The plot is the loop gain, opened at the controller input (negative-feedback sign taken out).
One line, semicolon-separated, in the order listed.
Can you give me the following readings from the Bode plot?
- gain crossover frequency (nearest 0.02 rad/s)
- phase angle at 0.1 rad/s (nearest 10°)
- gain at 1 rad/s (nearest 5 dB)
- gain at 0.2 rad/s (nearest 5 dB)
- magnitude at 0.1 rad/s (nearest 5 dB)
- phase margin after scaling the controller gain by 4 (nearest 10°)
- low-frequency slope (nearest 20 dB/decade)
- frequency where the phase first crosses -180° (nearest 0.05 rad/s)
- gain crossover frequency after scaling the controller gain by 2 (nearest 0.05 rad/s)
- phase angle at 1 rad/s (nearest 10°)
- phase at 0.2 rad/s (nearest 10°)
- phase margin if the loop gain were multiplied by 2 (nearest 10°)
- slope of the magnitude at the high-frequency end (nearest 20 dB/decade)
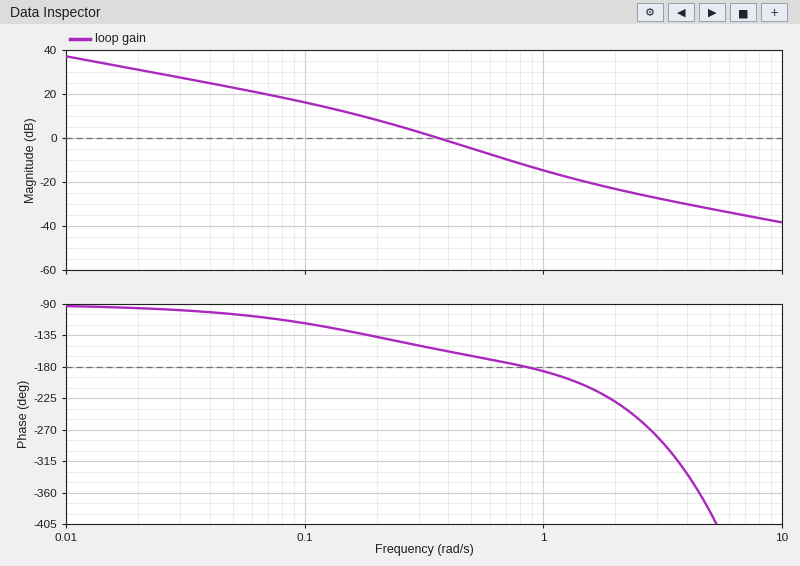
0.36 rad/s; -120°; -15 dB; 10 dB; 15 dB; 0°; -20 dB/decade; 0.85 rad/s; 0.55 rad/s; -190°; -140°; 10°; -20 dB/decade
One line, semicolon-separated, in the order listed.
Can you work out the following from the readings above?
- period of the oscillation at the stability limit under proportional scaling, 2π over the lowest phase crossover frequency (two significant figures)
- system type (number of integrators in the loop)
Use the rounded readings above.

7.4 s; 1
